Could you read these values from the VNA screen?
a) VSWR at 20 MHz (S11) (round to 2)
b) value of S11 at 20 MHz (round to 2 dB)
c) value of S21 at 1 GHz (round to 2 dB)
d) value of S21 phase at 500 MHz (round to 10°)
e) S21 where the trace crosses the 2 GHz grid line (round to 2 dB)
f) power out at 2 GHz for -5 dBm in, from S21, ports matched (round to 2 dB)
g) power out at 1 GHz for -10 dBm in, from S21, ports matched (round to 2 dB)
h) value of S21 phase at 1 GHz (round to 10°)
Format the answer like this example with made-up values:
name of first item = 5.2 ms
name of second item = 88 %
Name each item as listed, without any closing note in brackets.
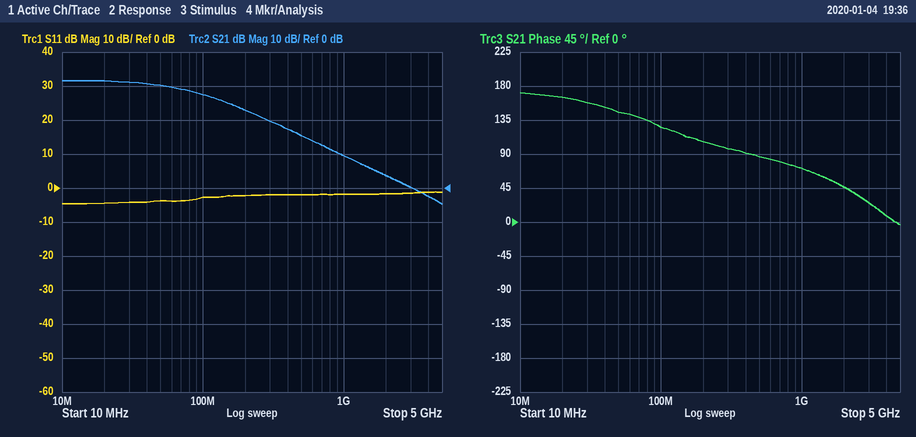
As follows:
VSWR at 20 MHz (S11) = 4
value of S11 at 20 MHz = -4 dB
value of S21 at 1 GHz = 10 dB
value of S21 phase at 500 MHz = 90°
S21 where the trace crosses the 2 GHz grid line = 4 dB
power out at 2 GHz for -5 dBm in, from S21, ports matched = -2 dBm
power out at 1 GHz for -10 dBm in, from S21, ports matched = 0 dBm
value of S21 phase at 1 GHz = 70°
